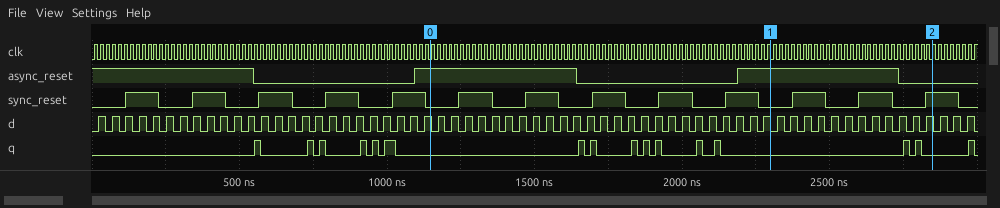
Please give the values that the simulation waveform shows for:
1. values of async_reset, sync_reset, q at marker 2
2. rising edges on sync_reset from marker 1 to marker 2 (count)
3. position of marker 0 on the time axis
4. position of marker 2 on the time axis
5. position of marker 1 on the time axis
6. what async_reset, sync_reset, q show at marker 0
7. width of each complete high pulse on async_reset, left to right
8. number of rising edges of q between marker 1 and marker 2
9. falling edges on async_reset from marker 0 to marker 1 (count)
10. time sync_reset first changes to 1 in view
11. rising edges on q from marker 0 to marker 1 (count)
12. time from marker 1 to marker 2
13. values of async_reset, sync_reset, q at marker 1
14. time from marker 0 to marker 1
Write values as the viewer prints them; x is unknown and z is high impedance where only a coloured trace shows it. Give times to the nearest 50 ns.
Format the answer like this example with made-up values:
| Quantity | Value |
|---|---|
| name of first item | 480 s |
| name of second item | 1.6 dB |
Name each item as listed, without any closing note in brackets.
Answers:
| Quantity | Value |
|---|---|
| values of async_reset, sync_reset, q at marker 2 | async_reset=0, sync_reset=1, q=0 |
| rising edges on sync_reset from marker 1 to marker 2 | 3 |
| position of marker 0 on the time axis | 1150 ns |
| position of marker 2 on the time axis | 2850 ns |
| position of marker 1 on the time axis | 2300 ns |
| what async_reset, sync_reset, q show at marker 0 | async_reset=1, sync_reset=0, q=0 |
| width of each complete high pulse on async_reset, left to right | 550 ns, 550 ns |
| number of rising edges of q between marker 1 and marker 2 | 2 |
| falling edges on async_reset from marker 0 to marker 1 | 1 |
| time sync_reset first changes to 1 in view | 100 ns |
| rising edges on q from marker 0 to marker 1 | 7 |
| time from marker 1 to marker 2 | 550 ns |
| values of async_reset, sync_reset, q at marker 1 | async_reset=1, sync_reset=0, q=0 |
| time from marker 0 to marker 1 | 1150 ns |
